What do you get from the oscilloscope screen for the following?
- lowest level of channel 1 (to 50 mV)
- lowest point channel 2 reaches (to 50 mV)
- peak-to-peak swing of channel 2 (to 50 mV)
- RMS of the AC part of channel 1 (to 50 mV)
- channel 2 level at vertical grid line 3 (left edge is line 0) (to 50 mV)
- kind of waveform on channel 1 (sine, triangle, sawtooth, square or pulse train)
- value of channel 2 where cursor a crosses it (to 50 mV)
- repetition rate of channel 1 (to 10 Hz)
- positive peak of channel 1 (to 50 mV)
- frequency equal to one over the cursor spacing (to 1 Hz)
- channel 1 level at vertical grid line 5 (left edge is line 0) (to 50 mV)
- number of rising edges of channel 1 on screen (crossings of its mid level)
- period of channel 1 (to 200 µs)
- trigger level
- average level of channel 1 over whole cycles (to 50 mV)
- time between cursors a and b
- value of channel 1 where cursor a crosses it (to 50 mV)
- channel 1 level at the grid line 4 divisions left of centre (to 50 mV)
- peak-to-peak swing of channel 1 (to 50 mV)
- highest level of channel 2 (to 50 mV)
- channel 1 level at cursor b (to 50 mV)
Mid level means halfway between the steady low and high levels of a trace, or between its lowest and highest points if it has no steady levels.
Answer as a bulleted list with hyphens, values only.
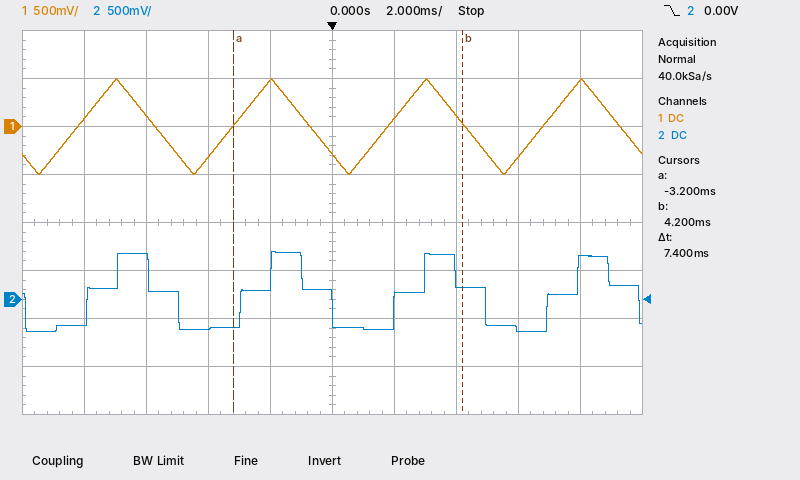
- -500 mV
- -350 mV
- 850 mV
- 300 mV
- -300 mV
- triangle
- -300 mV
- 200 Hz
- 500 mV
- 135 Hz
- -300 mV
- 4
- 5.0 ms
- 0.00 V
- 0 mV
- 7.4 ms
- 0 mV
- 100 mV
- 1.00 V
- 500 mV
- 50 mV
